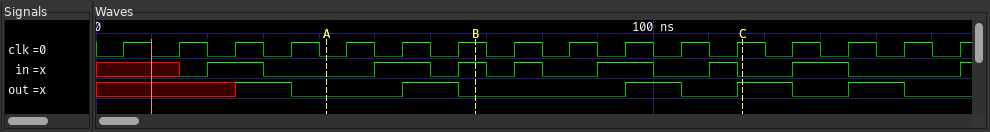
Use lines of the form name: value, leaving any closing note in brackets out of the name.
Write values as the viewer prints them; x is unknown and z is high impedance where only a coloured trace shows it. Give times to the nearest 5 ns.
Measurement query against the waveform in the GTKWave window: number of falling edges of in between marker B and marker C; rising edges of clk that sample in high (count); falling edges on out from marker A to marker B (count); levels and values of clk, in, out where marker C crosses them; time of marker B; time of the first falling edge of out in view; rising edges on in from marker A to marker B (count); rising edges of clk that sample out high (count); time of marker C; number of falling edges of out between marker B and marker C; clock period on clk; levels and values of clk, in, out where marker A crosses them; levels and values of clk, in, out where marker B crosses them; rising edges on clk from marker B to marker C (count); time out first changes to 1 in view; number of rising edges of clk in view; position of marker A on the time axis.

number of falling edges of in between marker B and marker C: 4
rising edges of clk that sample in high: 5
falling edges on out from marker A to marker B: 1
levels and values of clk, in, out where marker C crosses them: clk=1, in=0, out=1
time of marker B: 70 ns
time of the first falling edge of out in view: 35 ns
rising edges on in from marker A to marker B: 2
rising edges of clk that sample out high: 5
time of marker C: 115 ns
number of falling edges of out between marker B and marker C: 1
clock period on clk: 10 ns
levels and values of clk, in, out where marker A crosses them: clk=0, in=0, out=0
levels and values of clk, in, out where marker B crosses them: clk=1, in=1, out=0
rising edges on clk from marker B to marker C: 5
time out first changes to 1 in view: 25 ns
number of rising edges of clk in view: 16
position of marker A on the time axis: 40 ns
